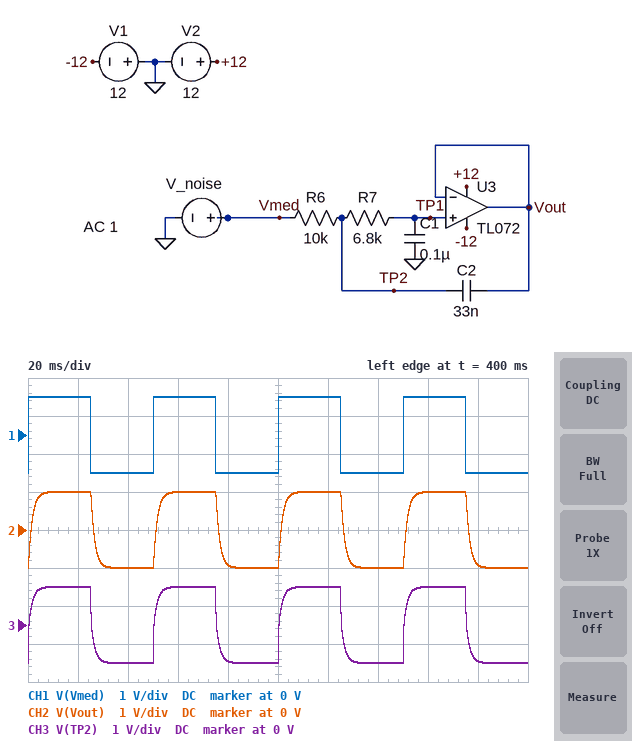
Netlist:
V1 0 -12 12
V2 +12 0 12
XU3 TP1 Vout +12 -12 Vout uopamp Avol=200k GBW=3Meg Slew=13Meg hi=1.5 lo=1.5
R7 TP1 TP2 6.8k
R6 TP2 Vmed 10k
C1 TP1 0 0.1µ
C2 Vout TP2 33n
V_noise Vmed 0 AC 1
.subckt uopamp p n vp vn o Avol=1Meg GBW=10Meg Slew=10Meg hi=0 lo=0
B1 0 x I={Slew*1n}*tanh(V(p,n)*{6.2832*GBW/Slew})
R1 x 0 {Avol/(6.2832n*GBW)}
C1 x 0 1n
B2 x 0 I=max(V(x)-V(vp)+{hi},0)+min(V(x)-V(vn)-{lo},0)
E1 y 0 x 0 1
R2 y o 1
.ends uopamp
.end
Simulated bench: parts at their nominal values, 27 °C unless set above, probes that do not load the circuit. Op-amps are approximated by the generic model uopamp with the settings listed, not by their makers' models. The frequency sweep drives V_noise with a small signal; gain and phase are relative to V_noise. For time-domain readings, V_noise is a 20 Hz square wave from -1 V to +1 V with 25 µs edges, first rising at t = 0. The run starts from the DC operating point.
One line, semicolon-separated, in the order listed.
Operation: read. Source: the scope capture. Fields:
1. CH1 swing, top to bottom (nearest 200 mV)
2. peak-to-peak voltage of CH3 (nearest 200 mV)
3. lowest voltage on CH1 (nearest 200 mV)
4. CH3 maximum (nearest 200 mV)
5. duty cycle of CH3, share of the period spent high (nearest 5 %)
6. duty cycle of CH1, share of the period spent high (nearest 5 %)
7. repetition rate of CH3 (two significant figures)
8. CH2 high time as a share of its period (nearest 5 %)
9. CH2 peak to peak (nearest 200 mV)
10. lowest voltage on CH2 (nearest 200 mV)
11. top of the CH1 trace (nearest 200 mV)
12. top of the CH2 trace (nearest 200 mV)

2.0 V; 2.0 V; -1.0 V; 1.0 V; 50 %; 50 %; 20 Hz; 50 %; 2.0 V; -1.0 V; 1.0 V; 1.0 V
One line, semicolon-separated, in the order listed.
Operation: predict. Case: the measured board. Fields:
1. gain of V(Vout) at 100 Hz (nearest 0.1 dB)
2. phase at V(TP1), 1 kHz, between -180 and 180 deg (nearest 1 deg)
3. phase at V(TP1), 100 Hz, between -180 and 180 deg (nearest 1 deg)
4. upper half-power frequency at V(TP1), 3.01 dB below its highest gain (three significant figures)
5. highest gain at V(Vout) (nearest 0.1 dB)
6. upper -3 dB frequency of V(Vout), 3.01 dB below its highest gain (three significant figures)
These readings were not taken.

-2.9 dB; -127 deg; -49 deg; 103 Hz; 0 dB; 103 Hz
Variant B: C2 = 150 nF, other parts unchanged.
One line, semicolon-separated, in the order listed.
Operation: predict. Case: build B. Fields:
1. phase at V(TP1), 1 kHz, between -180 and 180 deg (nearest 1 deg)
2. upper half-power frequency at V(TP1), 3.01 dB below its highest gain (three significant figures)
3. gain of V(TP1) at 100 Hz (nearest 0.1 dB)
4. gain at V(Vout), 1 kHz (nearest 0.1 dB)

-165 deg; 131 Hz; -1.7 dB; -32.2 dB
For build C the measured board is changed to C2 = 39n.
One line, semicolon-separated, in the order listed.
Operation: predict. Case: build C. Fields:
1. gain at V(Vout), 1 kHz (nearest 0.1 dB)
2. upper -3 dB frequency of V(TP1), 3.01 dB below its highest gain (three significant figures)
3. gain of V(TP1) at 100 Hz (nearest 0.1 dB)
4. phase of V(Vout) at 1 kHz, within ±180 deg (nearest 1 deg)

-23.0 dB; 104 Hz; -2.8 dB; -132 deg
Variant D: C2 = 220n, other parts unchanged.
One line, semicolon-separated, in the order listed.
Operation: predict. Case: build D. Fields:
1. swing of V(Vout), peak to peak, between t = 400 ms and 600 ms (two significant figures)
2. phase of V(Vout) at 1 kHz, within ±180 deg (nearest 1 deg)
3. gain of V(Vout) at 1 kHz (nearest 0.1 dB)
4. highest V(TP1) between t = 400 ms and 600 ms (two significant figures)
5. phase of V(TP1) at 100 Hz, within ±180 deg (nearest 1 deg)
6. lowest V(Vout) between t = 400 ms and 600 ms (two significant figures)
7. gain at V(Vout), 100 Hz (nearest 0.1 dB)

2.2 V; -170 deg; -35.4 dB; 1.1 V; -69 deg; -1.1 V; -1.1 dB
